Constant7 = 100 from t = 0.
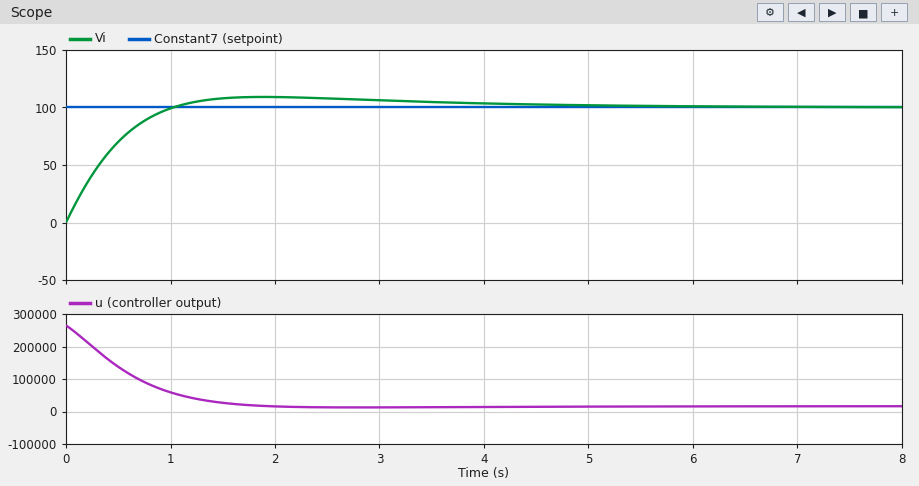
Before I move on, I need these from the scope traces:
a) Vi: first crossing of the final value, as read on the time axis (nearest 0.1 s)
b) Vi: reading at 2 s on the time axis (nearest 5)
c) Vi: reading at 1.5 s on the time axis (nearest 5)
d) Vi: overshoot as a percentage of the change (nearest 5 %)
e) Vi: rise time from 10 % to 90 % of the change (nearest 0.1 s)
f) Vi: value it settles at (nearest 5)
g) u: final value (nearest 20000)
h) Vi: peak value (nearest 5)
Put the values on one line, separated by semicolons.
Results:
1.0 s; 110; 110; 10 %; 0.7 s; 100; 20000; 110
